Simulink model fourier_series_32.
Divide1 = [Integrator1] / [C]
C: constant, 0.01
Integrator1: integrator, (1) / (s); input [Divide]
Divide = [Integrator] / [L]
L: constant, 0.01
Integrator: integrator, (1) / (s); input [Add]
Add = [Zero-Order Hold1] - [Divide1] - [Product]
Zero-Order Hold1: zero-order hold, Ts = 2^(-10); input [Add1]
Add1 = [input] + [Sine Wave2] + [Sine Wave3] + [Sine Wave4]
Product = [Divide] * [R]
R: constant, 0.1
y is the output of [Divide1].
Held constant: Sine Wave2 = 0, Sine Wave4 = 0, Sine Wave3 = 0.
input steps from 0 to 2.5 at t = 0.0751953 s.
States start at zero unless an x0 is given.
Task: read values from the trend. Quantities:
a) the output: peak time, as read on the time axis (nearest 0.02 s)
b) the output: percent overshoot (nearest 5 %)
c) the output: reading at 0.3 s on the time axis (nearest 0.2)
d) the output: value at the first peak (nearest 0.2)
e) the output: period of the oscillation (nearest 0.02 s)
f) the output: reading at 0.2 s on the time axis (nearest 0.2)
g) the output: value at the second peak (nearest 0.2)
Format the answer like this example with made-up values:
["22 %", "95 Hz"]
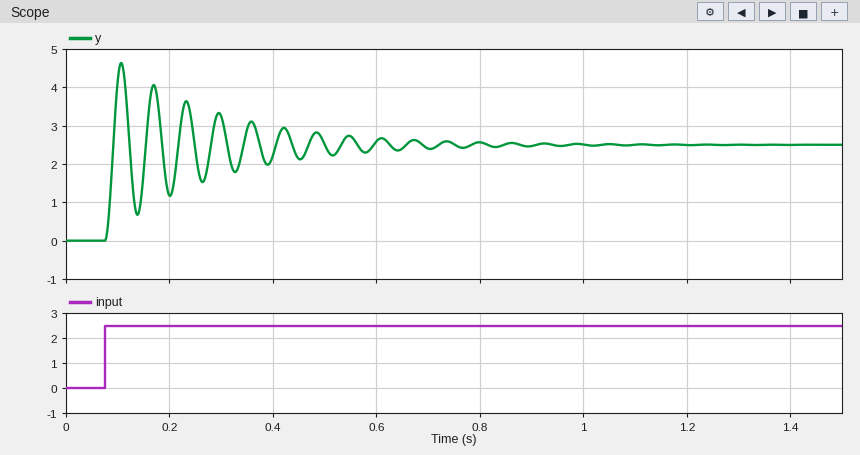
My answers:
["0.10 s", "85 %", "3.2", "4.6", "0.06 s", "1.2", "4.0"]
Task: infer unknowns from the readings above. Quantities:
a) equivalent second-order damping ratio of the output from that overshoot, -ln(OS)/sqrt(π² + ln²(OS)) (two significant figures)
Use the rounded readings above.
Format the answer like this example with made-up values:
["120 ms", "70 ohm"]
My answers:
["0.052"]
